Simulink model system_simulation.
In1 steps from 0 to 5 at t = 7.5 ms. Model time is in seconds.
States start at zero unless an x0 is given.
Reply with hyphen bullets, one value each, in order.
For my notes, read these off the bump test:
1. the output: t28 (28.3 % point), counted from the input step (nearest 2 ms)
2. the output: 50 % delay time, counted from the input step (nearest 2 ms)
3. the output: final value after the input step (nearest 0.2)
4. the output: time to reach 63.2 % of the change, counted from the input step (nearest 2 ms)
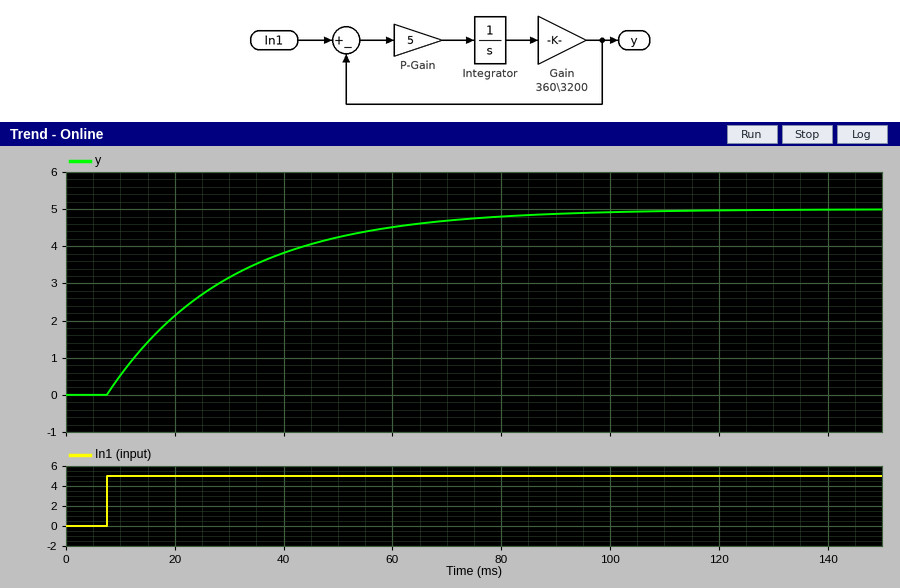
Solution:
- 8 ms
- 16 ms
- 5.0
- 22 ms
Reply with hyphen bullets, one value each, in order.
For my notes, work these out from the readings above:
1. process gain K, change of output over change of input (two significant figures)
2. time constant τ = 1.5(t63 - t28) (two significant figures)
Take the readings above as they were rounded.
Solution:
- 1.0
- 21 ms
